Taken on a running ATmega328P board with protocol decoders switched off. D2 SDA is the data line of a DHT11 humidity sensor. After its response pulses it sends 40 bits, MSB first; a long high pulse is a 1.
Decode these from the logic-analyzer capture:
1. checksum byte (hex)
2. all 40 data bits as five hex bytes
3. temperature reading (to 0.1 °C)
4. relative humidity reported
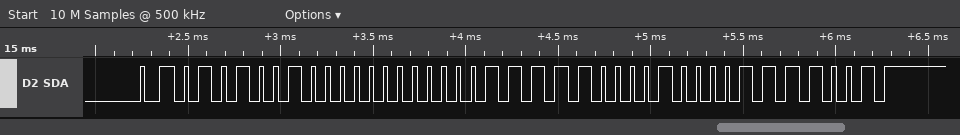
0x79
52 00 1F 08 79
31.8 °C
82 %
